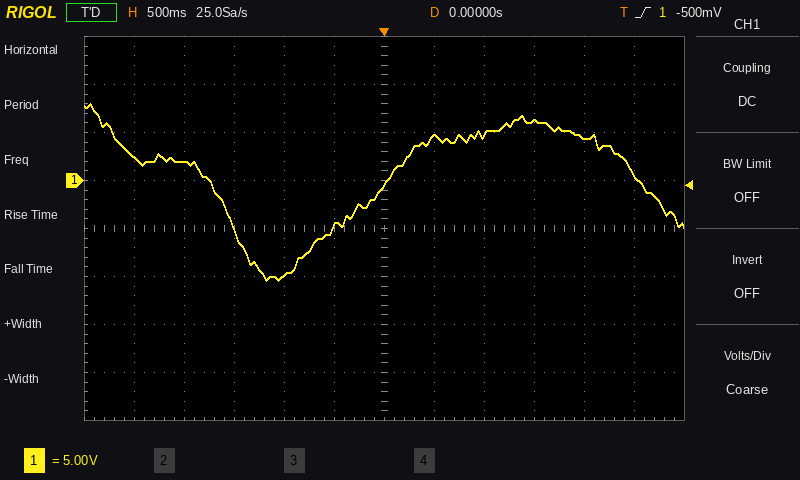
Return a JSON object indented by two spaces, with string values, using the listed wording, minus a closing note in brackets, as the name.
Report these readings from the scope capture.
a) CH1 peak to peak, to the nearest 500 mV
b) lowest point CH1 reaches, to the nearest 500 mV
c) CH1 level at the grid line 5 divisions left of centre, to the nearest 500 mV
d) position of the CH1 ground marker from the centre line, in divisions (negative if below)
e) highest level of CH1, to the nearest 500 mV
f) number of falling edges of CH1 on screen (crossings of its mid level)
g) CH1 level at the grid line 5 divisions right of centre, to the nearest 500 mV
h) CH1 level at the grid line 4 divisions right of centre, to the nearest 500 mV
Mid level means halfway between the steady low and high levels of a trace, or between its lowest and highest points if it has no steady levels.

{
  "CH1 peak to peak, to the nearest 500 mV": "18.5 V",
  "lowest point CH1 reaches, to the nearest 500 mV": "-10.5 V",
  "CH1 level at the grid line 5 divisions left of centre, to the nearest 500 mV": "2.5 V",
  "position of the CH1 ground marker from the centre line, in divisions": "+1.0 div",
  "highest level of CH1, to the nearest 500 mV": "8.0 V",
  "number of falling edges of CH1 on screen": "2",
  "CH1 level at the grid line 5 divisions right of centre, to the nearest 500 mV": "500 mV",
  "CH1 level at the grid line 4 divisions right of centre, to the nearest 500 mV": "4.5 V"
}
